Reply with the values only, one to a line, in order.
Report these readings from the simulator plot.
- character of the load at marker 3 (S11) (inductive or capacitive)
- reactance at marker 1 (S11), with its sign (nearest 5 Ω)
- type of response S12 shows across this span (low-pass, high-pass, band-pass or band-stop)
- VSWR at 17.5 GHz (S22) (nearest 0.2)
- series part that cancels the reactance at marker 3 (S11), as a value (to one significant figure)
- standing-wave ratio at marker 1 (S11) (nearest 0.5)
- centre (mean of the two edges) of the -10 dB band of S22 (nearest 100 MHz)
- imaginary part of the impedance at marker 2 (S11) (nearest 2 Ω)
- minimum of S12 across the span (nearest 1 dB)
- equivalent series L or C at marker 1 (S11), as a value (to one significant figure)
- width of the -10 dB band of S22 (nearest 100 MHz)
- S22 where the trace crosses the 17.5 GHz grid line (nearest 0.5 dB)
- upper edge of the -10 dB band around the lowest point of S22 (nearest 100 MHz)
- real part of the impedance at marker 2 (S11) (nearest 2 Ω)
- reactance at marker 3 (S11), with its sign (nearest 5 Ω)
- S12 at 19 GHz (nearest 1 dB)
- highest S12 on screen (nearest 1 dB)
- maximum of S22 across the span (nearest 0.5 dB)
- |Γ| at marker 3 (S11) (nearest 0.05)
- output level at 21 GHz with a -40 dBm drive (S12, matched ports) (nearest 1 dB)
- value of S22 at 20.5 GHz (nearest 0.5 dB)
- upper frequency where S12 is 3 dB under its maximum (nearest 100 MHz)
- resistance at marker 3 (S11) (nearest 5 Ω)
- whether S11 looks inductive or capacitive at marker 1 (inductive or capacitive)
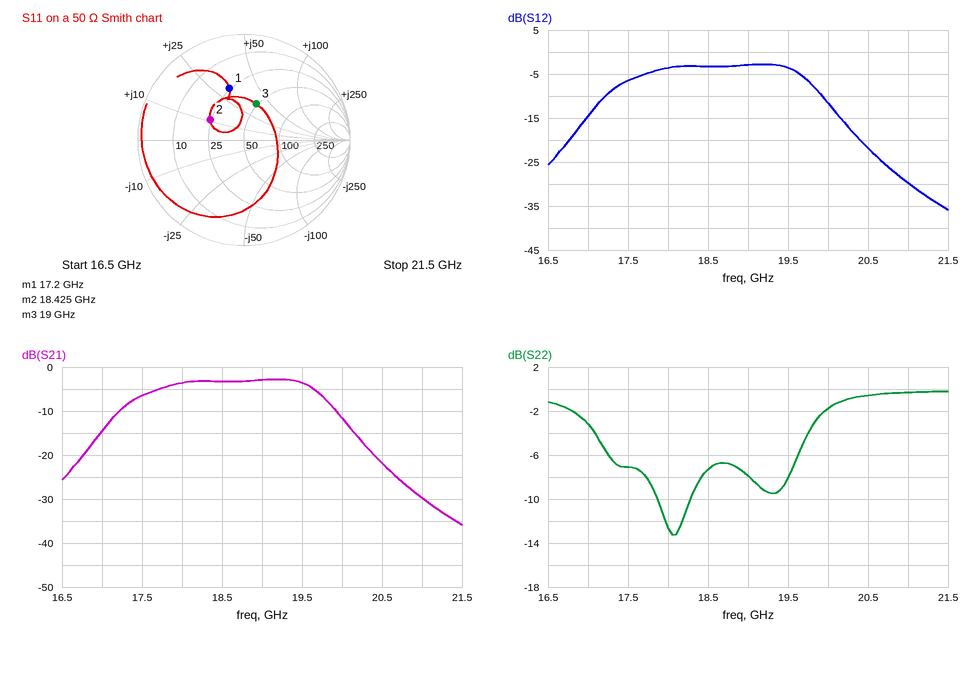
inductive
+30 Ω
band-pass
2.6
200 fF
3.0
18.1 GHz
+10 Ω
-36 dB
300 pH
400 MHz
-7.0 dB
18.3 GHz
24 Ω
+40 Ω
-3 dB
-3 dB
0.0 dB
0.35
-70 dBm
-0.5 dB
19.7 GHz
50 Ω
inductive
